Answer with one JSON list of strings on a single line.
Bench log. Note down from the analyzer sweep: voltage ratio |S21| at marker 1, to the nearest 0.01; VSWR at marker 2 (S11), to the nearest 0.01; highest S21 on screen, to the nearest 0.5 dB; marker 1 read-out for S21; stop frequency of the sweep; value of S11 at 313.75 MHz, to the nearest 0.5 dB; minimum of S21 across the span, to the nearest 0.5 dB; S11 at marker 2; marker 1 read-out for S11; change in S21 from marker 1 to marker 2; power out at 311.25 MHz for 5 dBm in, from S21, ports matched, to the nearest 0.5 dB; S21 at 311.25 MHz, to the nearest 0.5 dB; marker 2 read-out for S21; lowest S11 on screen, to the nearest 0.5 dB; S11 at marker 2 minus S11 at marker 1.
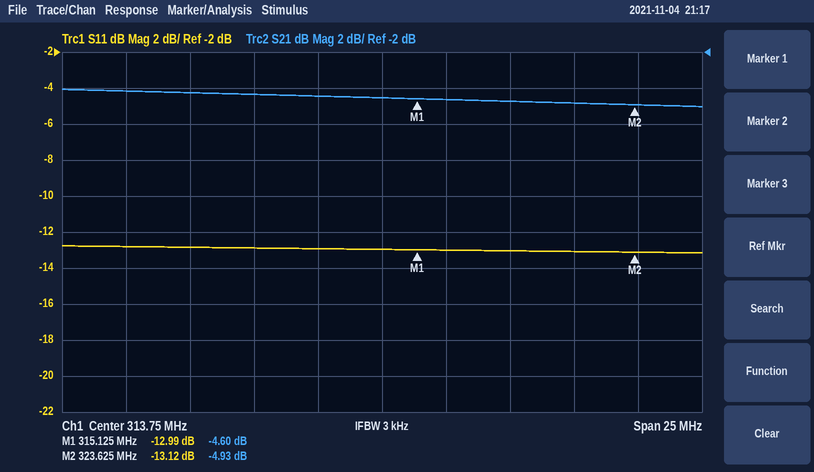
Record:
["0.59", "1.57", "-4.0 dB", "-4.60 dB", "326.25 MHz", "-13.0 dB", "-5.0 dB", "-13.12 dB", "-12.99 dB", "-0.33 dB", "0.5 dBm", "-4.5 dB", "-4.93 dB", "-13.0 dB", "-0.13 dB"]
